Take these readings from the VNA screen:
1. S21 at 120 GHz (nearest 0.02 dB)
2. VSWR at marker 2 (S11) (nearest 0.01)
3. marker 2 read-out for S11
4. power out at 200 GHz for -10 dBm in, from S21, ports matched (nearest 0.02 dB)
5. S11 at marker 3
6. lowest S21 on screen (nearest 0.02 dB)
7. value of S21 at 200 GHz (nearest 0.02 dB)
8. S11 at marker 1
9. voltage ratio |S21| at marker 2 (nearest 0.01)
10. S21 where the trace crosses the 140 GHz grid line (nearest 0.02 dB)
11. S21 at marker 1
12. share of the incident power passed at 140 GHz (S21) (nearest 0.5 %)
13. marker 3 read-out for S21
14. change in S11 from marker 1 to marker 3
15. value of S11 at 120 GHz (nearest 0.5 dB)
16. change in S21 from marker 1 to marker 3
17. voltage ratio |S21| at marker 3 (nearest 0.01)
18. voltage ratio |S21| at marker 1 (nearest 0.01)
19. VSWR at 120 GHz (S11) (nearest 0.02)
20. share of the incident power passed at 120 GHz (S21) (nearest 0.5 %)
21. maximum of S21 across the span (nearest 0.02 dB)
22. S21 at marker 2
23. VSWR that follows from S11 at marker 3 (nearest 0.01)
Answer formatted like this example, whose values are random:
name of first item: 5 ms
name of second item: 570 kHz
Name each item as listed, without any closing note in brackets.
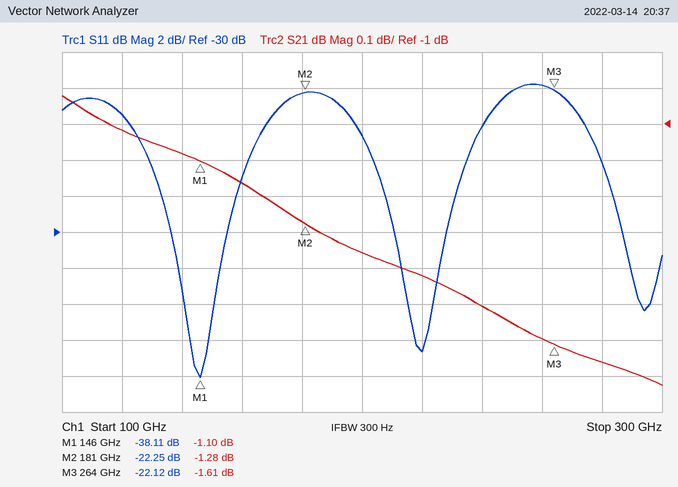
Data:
S21 at 120 GHz: -1.02 dB
VSWR at marker 2 (S11): 1.17
marker 2 read-out for S11: -22.25 dB
power out at 200 GHz for -10 dBm in, from S21, ports matched: -11.36 dBm
S11 at marker 3: -22.12 dB
lowest S21 on screen: -1.72 dB
value of S21 at 200 GHz: -1.36 dB
S11 at marker 1: -38.11 dB
voltage ratio |S21| at marker 2: 0.86
S21 where the trace crosses the 140 GHz grid line: -1.08 dB
S21 at marker 1: -1.10 dB
share of the incident power passed at 140 GHz (S21): 78.0 %
marker 3 read-out for S21: -1.61 dB
change in S11 from marker 1 to marker 3: 15.99 dB
value of S11 at 120 GHz: -23.5 dB
change in S21 from marker 1 to marker 3: -0.51 dB
voltage ratio |S21| at marker 3: 0.83
voltage ratio |S21| at marker 1: 0.88
VSWR at 120 GHz (S11): 1.14
share of the incident power passed at 120 GHz (S21): 79.0 %
maximum of S21 across the span: -0.92 dB
S21 at marker 2: -1.28 dB
VSWR that follows from S11 at marker 3: 1.17
